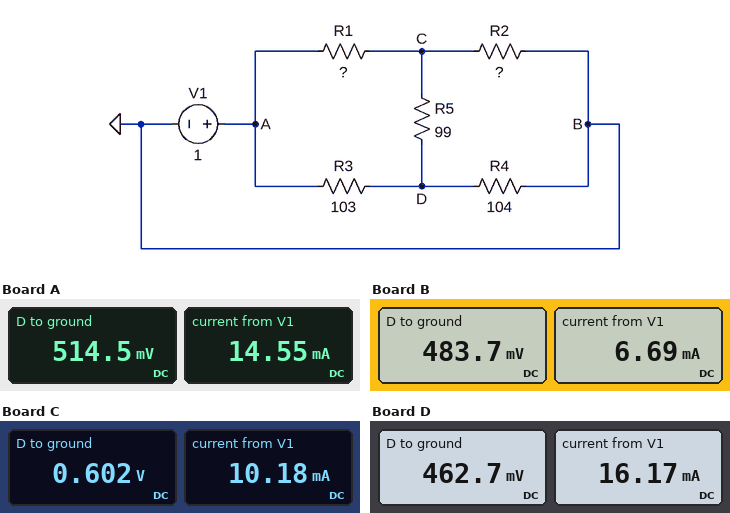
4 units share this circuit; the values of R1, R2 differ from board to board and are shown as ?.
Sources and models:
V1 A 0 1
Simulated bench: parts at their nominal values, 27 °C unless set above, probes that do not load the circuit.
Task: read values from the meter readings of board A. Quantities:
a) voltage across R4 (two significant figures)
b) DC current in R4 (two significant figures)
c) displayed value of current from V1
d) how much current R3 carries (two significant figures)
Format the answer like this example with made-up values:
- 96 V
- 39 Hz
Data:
- 510 mV
- 4.9 mA
- 14.55 mA
- 4.7 mA
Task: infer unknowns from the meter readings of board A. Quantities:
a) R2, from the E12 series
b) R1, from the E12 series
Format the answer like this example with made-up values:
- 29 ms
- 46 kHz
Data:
- 56 Ω
- 47 Ω
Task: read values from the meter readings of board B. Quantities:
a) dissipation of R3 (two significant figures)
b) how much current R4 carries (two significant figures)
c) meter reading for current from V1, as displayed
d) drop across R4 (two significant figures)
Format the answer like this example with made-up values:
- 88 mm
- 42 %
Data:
- 2.6 mW
- 4.7 mA
- 6.69 mA
- 480 mV
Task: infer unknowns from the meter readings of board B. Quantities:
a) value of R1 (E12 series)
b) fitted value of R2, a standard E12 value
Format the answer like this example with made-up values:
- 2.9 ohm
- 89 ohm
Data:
- 330 Ω
- 220 Ω
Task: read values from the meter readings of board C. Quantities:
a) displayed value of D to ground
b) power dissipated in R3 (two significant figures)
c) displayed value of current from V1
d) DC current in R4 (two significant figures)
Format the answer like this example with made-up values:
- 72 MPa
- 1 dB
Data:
- 0.602 V
- 1.5 mW
- 10.18 mA
- 5.8 mA
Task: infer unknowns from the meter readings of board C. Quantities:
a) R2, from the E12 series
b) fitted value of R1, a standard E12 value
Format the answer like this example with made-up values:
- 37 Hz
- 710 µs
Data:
- 180 Ω
- 33 Ω
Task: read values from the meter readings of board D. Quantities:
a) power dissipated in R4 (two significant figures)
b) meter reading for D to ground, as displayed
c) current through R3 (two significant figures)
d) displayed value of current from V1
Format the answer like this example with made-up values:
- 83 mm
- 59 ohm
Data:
- 2.1 mW
- 462.7 mV
- 5.2 mA
- 16.17 mA
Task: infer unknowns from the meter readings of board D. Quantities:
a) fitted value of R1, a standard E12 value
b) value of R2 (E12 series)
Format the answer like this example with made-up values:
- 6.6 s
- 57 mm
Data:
- 56 Ω
- 33 Ω
